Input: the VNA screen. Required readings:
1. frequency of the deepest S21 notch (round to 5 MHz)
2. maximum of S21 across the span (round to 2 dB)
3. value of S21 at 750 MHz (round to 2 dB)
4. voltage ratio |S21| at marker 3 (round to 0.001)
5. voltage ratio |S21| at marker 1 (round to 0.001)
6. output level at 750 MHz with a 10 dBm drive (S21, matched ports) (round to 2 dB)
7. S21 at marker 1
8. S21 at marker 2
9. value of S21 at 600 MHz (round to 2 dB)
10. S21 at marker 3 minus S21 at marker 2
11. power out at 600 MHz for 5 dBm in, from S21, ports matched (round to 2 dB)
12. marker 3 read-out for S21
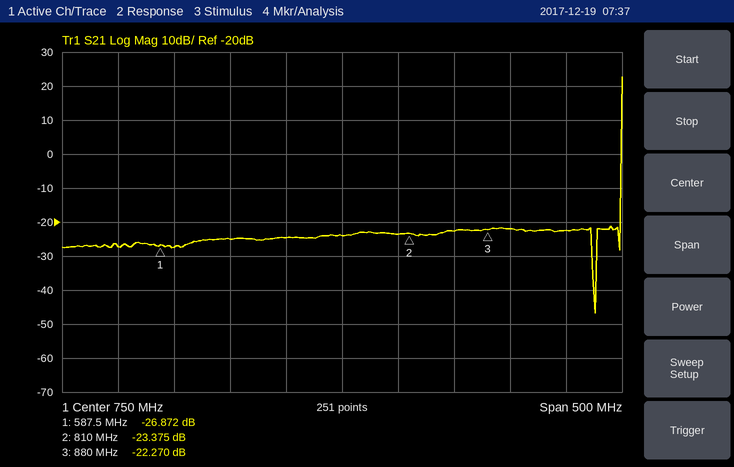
975 MHz
22 dB
-24 dB
0.077
0.045
-14 dBm
-26.872 dB
-23.375 dB
-28 dB
1.105 dB
-22 dBm
-22.270 dB
